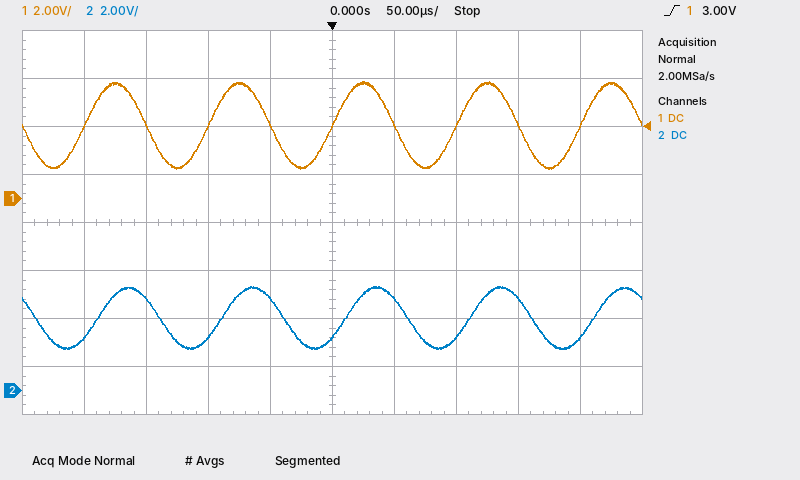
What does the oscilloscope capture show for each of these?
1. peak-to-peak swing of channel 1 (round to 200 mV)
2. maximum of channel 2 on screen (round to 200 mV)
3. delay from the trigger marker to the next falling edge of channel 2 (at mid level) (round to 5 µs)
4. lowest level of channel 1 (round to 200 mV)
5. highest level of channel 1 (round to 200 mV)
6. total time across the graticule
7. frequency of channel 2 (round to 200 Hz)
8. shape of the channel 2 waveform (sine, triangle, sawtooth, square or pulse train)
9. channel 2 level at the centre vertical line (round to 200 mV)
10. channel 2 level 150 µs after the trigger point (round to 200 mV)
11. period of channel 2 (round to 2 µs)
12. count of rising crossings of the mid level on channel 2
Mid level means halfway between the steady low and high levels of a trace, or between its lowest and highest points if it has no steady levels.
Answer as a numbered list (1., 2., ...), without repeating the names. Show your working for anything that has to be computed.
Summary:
1. 4.8 V − (1.2 V) = 3.6 V
2. 4.4 V
3. 60 µs
4. 1.2 V
5. 4.8 V
6. 500 µs
7. 1 / 100 µs ≈ 10.0 kHz
8. sine
9. 2.2 V
10. 3.8 V
11. 100 µs
12. 5
